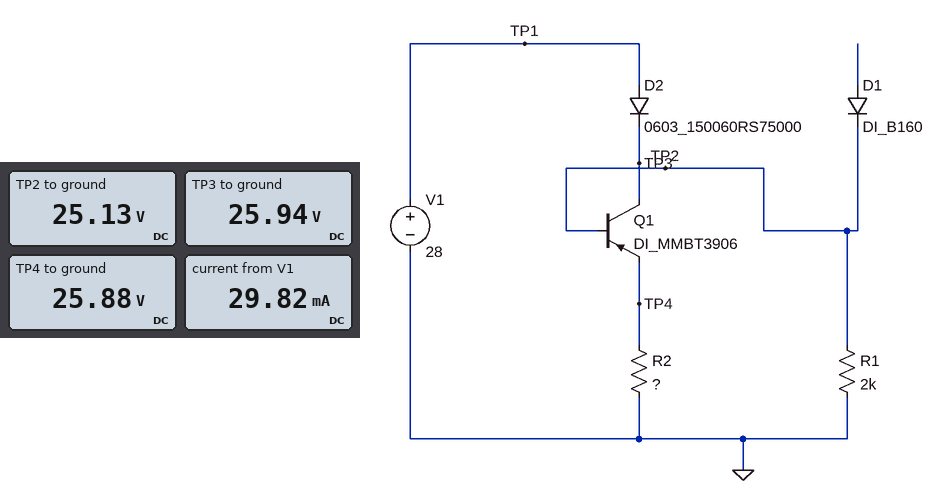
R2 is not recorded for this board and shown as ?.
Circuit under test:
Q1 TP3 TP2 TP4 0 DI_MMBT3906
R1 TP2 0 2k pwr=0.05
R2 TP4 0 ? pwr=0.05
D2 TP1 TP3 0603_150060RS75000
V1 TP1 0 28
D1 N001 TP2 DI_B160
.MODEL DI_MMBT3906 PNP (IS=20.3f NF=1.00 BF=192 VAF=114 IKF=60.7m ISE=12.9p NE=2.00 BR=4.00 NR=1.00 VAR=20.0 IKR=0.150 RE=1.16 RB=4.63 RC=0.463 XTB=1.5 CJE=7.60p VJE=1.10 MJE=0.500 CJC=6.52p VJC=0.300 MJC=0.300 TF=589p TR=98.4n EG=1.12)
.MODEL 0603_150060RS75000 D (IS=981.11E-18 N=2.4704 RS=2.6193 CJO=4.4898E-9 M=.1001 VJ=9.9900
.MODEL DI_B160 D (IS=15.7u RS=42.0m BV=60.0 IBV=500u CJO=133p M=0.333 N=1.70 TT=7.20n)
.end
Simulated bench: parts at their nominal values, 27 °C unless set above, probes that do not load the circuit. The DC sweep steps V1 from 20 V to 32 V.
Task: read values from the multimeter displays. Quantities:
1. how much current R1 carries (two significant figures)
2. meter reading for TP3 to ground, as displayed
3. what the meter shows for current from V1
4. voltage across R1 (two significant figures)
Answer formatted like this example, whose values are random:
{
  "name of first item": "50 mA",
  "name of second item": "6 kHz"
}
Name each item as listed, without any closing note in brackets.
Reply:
{
  "how much current R1 carries": "13 mA",
  "meter reading for TP3 to ground, as displayed": "25.94 V",
  "what the meter shows for current from V1": "29.82 mA",
  "voltage across R1": "25 V"
}
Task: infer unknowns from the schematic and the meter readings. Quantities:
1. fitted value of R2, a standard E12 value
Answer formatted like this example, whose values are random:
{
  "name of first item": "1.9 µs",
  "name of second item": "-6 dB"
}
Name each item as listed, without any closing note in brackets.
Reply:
{
  "fitted value of R2, a standard E12 value": "1.5 kΩ"
}
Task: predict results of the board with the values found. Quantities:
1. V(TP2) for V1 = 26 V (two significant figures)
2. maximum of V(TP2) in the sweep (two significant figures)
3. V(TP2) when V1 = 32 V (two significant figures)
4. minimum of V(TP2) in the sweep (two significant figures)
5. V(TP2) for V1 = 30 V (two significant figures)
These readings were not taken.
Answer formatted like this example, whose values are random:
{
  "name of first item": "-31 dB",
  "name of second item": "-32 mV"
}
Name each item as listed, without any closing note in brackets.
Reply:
{
  "V(TP2) for V1 = 26 V": "23 V",
  "maximum of V(TP2) in the sweep": "29 V",
  "V(TP2) when V1 = 32 V": "29 V",
  "minimum of V(TP2) in the sweep": "17 V",
  "V(TP2) for V1 = 30 V": "27 V"
}
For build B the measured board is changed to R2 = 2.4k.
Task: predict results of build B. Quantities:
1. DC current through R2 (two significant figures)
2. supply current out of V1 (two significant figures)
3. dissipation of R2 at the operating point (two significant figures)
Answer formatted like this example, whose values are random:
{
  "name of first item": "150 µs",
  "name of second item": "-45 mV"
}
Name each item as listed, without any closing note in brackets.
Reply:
{
  "DC current through R2": "11 mA",
  "supply current out of V1": "23 mA",
  "dissipation of R2 at the operating point": "280 mW"
}
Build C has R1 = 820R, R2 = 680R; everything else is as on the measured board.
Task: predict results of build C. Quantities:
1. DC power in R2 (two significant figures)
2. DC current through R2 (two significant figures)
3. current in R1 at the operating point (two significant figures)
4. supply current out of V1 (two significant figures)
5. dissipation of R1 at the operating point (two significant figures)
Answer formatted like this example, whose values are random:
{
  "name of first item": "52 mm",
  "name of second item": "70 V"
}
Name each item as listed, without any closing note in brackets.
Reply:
{
  "DC power in R2": "970 mW",
  "DC current through R2": "38 mA",
  "current in R1 at the operating point": "30 mA",
  "supply current out of V1": "68 mA",
  "dissipation of R1 at the operating point": "750 mW"
}
